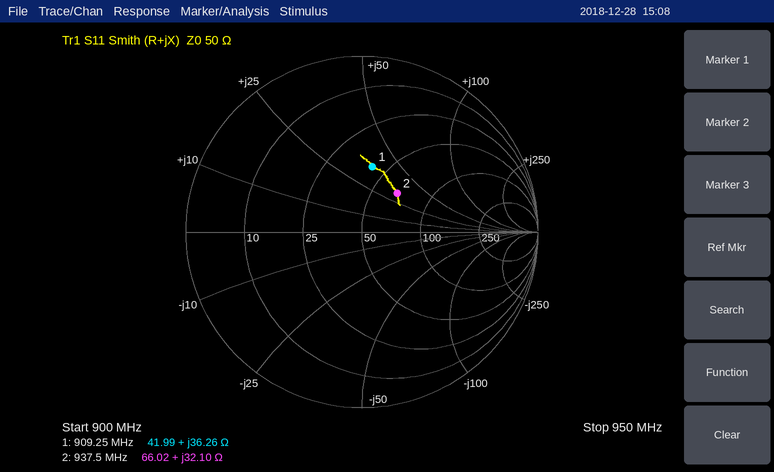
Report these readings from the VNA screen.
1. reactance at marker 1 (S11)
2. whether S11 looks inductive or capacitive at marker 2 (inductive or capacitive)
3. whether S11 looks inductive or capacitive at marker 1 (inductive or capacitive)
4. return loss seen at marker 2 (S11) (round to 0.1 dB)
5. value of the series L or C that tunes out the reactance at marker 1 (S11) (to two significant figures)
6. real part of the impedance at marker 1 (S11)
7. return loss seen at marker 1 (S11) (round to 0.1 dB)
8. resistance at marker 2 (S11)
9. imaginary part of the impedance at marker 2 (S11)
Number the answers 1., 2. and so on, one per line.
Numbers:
1. +36.26 Ω
2. inductive
3. inductive
4. 10.5 dB
5. 4.8 pF
6. 41.99 Ω
7. 8.5 dB
8. 66.02 Ω
9. +32.10 Ω
